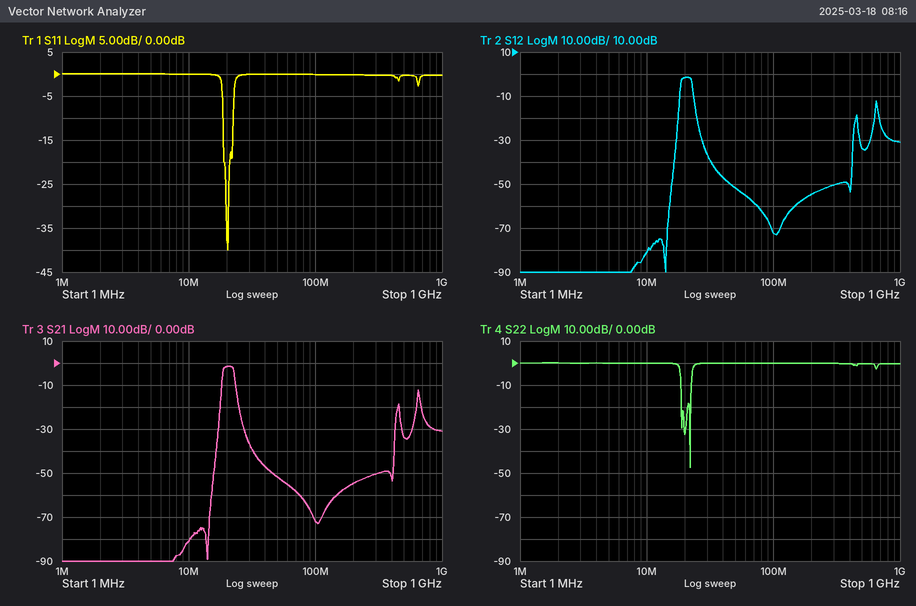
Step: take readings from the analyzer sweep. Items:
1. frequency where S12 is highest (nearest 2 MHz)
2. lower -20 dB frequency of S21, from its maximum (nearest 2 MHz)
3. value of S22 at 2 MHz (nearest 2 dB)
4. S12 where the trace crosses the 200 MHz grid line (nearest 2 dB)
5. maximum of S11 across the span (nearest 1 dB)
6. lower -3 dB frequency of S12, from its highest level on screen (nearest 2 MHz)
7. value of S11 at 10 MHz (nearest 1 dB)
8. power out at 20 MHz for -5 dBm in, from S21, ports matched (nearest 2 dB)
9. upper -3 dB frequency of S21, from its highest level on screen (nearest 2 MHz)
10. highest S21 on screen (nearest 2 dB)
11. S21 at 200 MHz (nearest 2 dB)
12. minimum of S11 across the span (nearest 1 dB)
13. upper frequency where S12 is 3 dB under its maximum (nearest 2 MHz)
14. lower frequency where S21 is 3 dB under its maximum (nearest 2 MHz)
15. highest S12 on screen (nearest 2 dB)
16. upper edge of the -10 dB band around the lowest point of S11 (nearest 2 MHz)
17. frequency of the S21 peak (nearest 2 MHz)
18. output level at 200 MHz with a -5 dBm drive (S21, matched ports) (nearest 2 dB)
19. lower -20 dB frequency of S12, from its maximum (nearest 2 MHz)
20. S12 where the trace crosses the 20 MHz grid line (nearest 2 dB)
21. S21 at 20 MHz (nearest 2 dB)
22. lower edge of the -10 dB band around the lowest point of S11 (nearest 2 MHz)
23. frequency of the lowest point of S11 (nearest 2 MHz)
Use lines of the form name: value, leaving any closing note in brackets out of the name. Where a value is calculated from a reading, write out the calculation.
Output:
frequency where S12 is highest: 20 MHz
lower -20 dB frequency of S21, from its maximum: 18 MHz
value of S22 at 2 MHz: 0 dB
S12 where the trace crosses the 200 MHz grid line: -54 dB
maximum of S11 across the span: 0 dB
lower -3 dB frequency of S12, from its highest level on screen: 18 MHz
value of S11 at 10 MHz: 0 dB
power out at 20 MHz for -5 dBm in, from S21, ports matched: -5 dBm + (-2 dB) = -6 dBm
upper -3 dB frequency of S21, from its highest level on screen: 22 MHz
highest S21 on screen: -2 dB
S21 at 200 MHz: -54 dB
minimum of S11 across the span: -40 dB
upper frequency where S12 is 3 dB under its maximum: 22 MHz
lower frequency where S21 is 3 dB under its maximum: 18 MHz
highest S12 on screen: -2 dB
upper edge of the -10 dB band around the lowest point of S11: 22 MHz
frequency of the S21 peak: 20 MHz
output level at 200 MHz with a -5 dBm drive (S21, matched ports): -5 dBm + (-54 dB) = -60 dBm
lower -20 dB frequency of S12, from its maximum: 18 MHz
S12 where the trace crosses the 20 MHz grid line: -2 dB
S21 at 20 MHz: -2 dB
lower edge of the -10 dB band around the lowest point of S11: 18 MHz
frequency of the lowest point of S11: 20 MHz
